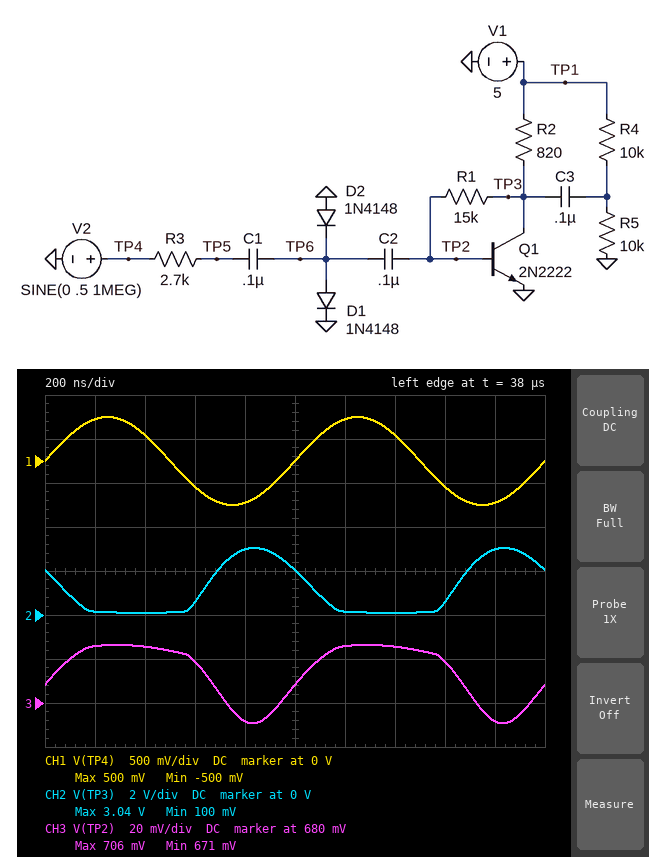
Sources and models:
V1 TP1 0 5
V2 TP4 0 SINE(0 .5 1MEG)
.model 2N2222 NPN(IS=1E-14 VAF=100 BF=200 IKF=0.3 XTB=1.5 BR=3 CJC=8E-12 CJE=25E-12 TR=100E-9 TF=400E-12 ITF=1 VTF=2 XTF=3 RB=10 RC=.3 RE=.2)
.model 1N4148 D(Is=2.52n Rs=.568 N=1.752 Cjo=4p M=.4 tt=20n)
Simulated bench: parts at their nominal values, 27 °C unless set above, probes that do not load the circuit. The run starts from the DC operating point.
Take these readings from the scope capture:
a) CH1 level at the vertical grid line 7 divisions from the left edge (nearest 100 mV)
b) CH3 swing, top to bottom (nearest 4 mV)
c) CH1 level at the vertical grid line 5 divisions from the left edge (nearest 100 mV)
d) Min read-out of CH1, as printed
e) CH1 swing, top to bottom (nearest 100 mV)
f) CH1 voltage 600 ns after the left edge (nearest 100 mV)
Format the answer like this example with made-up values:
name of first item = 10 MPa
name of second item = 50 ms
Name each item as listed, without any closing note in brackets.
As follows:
CH1 level at the vertical grid line 7 divisions from the left edge = 300 mV
CH3 swing, top to bottom = 36 mV
CH1 level at the vertical grid line 5 divisions from the left edge = 0 V
Min read-out of CH1, as printed = -500 mV
CH1 swing, top to bottom = 1.0 V
CH1 voltage 600 ns after the left edge = -300 mV
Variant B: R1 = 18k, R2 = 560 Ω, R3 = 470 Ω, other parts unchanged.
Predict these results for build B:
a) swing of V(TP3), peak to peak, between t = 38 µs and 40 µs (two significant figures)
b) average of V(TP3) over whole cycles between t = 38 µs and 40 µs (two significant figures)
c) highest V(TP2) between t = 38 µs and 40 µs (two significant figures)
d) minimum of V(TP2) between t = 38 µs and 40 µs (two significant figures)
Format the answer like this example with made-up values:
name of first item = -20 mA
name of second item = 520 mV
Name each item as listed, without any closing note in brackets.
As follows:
swing of V(TP3), peak to peak, between t = 38 µs and 40 µs = 4.5 V
average of V(TP3) over whole cycles between t = 38 µs and 40 µs = 2.0 V
highest V(TP2) between t = 38 µs and 40 µs = 730 mV
minimum of V(TP2) between t = 38 µs and 40 µs = 250 mV
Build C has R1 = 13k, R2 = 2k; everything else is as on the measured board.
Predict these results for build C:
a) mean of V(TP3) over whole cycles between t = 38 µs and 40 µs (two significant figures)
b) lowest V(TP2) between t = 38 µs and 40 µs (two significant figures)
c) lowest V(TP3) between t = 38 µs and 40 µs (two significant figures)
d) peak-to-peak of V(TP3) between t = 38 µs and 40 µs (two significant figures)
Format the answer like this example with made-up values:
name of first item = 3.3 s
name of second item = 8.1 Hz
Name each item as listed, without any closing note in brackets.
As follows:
mean of V(TP3) over whole cycles between t = 38 µs and 40 µs = 980 mV
lowest V(TP2) between t = 38 µs and 40 µs = 640 mV
lowest V(TP3) between t = 38 µs and 40 µs = 77 mV
peak-to-peak of V(TP3) between t = 38 µs and 40 µs = 2.6 V
